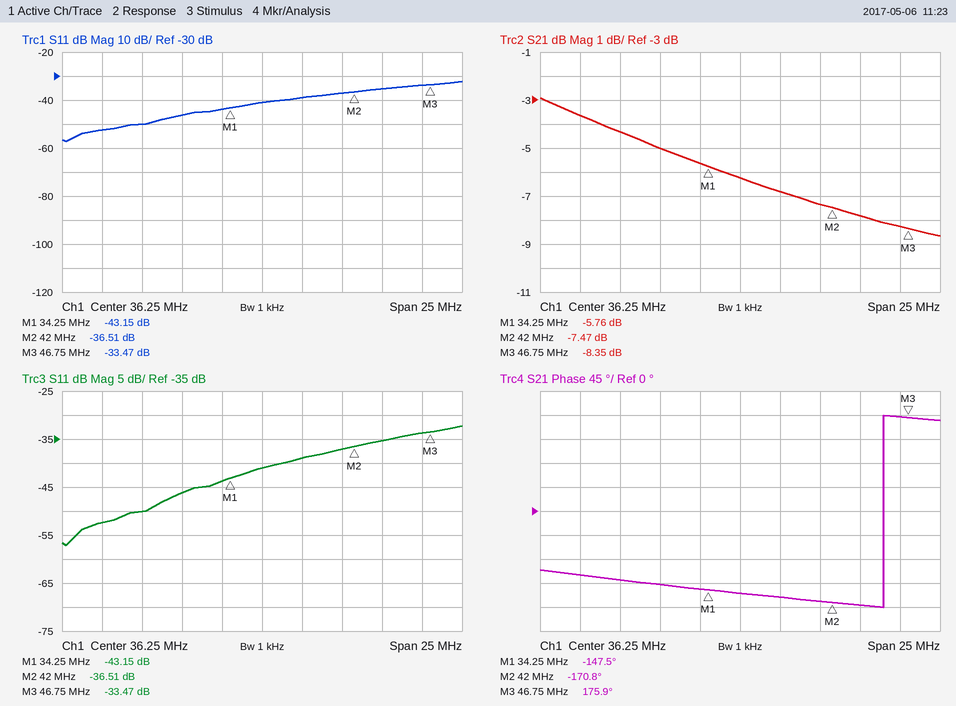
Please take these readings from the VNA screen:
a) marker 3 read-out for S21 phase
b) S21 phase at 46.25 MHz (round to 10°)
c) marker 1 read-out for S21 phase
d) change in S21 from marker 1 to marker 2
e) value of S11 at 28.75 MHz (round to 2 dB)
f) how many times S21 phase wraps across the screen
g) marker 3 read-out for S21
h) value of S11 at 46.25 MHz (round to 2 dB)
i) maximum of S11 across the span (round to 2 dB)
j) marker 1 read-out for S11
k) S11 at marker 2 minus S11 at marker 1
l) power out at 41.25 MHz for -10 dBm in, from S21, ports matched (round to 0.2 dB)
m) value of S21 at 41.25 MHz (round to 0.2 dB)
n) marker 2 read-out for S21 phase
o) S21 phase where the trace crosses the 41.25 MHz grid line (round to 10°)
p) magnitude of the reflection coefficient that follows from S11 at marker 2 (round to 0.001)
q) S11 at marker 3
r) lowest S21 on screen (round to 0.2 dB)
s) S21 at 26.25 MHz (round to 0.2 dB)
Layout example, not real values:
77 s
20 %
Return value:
175.9°
180°
-147.5°
-1.71 dB
-50 dB
1
-8.35 dB
-34 dB
-32 dB
-43.15 dB
6.64 dB
-17.4 dBm
-7.4 dB
-170.8°
-170°
0.015
-33.47 dB
-8.6 dB
-3.6 dB
